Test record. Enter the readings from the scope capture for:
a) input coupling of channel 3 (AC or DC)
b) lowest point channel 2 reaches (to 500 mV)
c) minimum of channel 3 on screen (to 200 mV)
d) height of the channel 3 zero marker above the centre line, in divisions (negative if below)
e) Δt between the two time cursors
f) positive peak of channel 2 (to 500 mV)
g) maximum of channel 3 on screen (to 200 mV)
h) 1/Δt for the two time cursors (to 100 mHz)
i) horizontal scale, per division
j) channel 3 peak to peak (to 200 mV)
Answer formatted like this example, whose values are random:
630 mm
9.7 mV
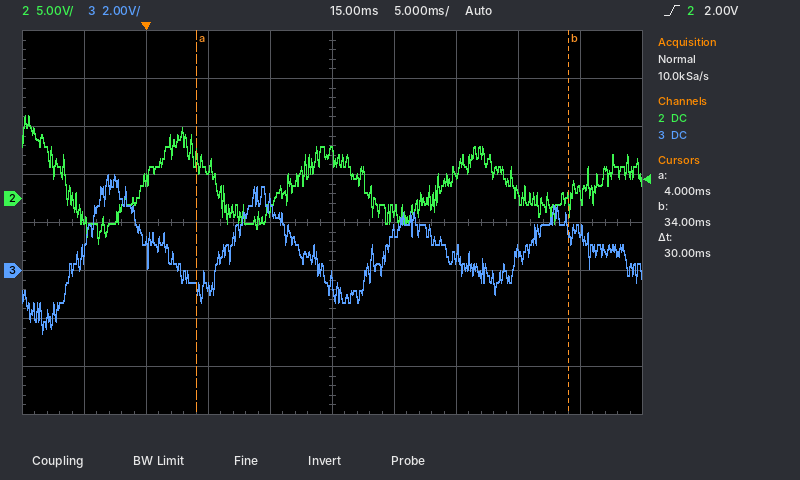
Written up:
DC
-4.5 V
-2.6 V
-1.0 div
30 ms
8.5 V
4.0 V
33.3 Hz
5 ms
6.6 V
